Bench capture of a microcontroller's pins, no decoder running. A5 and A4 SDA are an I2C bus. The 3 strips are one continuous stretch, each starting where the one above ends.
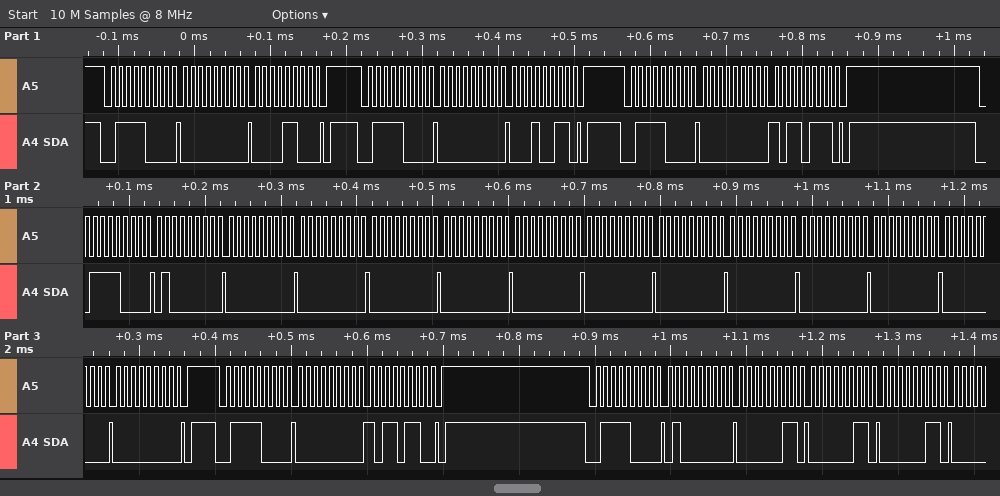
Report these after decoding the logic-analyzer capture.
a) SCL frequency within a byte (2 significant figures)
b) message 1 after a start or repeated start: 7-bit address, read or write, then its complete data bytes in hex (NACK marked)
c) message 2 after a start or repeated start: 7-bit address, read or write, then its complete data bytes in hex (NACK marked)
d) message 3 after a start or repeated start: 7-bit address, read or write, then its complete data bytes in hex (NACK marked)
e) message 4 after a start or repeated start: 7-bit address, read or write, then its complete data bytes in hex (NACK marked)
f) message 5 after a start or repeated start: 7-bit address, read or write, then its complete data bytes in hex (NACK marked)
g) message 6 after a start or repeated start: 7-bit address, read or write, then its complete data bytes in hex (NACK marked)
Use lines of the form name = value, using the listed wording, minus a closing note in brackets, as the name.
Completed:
SCL frequency within a byte = 100 kHz
message 1 after a start or repeated start: 7-bit address, read or write, then its complete data bytes in hex = 0x3C write: 00 0C
message 2 after a start or repeated start: 7-bit address, read or write, then its complete data bytes in hex = 0x3C write: 00 13
message 3 after a start or repeated start: 7-bit address, read or write, then its complete data bytes in hex = 0x3C write: 00 B7
message 4 after a start or repeated start: 7-bit address, read or write, then its complete data bytes in hex = 0x3C write: 40 00 00 00 00 00 00 00 00 00 00 00 00
message 5 after a start or repeated start: 7-bit address, read or write, then its complete data bytes in hex = 0x3C write: 00 B6
message 6 after a start or repeated start: 7-bit address, read or write, then its complete data bytes in hex = 0x3C write: 40 03 03 03
